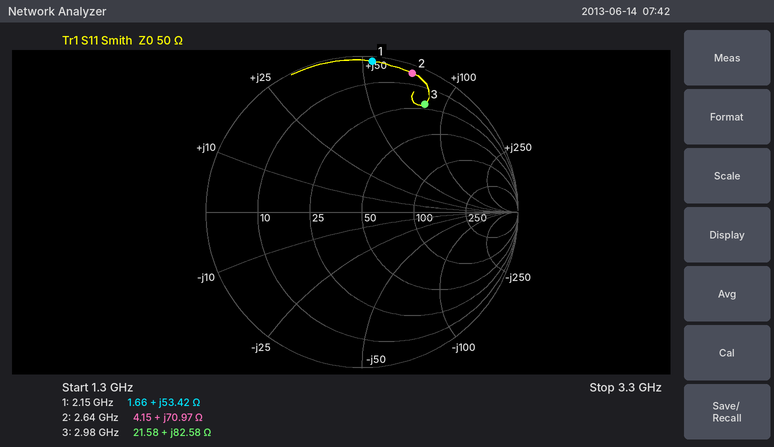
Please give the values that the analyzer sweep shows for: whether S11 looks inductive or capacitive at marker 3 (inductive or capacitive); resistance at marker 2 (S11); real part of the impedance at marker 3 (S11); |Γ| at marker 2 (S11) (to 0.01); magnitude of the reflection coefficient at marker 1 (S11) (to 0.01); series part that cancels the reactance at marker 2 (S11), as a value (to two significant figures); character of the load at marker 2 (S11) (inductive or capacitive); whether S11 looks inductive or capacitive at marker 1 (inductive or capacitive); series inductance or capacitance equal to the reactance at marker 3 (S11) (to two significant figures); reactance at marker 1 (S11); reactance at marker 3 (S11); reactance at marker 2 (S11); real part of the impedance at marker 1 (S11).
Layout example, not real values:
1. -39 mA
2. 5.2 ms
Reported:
1. inductive
2. 4.15 Ω
3. 21.58 Ω
4. 0.95
5. 0.97
6. 850 fF
7. inductive
8. inductive
9. 4.4 nH
10. +53.42 Ω
11. +82.58 Ω
12. +70.97 Ω
13. 1.66 Ω
